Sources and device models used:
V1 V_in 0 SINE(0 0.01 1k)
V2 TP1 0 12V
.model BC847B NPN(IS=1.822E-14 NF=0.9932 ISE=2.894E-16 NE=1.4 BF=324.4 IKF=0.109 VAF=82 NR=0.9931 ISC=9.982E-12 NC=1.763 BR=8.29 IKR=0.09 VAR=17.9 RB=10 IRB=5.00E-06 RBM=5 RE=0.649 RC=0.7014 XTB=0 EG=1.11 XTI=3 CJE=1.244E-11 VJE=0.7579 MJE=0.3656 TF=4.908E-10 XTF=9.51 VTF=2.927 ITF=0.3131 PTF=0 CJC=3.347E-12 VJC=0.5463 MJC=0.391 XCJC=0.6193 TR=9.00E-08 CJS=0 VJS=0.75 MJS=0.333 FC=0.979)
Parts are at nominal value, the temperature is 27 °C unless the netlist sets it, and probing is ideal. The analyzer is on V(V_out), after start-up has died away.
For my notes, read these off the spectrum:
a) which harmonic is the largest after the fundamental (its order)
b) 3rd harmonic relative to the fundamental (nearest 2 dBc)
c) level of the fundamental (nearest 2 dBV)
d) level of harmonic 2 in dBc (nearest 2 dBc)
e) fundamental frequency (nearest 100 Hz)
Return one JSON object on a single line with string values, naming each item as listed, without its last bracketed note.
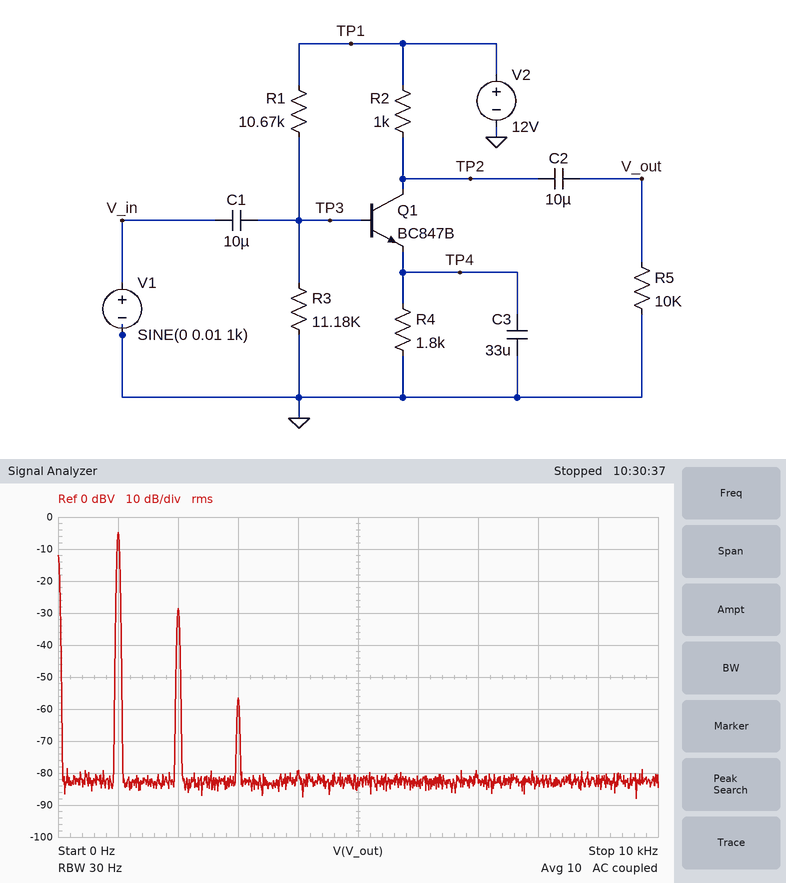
{"which harmonic is the largest after the fundamental": "2", "3rd harmonic relative to the fundamental": "-52 dBc", "level of the fundamental": "-4 dBV", "level of harmonic 2 in dBc": "-24 dBc", "fundamental frequency": "1.0 kHz"}
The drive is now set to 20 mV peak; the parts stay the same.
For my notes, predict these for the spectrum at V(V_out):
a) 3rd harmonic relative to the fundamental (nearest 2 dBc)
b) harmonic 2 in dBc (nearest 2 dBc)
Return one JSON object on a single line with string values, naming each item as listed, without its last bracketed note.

{"3rd harmonic relative to the fundamental": "-40 dBc", "harmonic 2 in dBc": "-18 dBc"}
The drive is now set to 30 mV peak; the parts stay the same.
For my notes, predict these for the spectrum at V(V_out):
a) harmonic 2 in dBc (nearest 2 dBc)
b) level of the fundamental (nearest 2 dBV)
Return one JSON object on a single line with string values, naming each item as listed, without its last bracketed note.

{"harmonic 2 in dBc": "-14 dBc", "level of the fundamental": "4 dBV"}
